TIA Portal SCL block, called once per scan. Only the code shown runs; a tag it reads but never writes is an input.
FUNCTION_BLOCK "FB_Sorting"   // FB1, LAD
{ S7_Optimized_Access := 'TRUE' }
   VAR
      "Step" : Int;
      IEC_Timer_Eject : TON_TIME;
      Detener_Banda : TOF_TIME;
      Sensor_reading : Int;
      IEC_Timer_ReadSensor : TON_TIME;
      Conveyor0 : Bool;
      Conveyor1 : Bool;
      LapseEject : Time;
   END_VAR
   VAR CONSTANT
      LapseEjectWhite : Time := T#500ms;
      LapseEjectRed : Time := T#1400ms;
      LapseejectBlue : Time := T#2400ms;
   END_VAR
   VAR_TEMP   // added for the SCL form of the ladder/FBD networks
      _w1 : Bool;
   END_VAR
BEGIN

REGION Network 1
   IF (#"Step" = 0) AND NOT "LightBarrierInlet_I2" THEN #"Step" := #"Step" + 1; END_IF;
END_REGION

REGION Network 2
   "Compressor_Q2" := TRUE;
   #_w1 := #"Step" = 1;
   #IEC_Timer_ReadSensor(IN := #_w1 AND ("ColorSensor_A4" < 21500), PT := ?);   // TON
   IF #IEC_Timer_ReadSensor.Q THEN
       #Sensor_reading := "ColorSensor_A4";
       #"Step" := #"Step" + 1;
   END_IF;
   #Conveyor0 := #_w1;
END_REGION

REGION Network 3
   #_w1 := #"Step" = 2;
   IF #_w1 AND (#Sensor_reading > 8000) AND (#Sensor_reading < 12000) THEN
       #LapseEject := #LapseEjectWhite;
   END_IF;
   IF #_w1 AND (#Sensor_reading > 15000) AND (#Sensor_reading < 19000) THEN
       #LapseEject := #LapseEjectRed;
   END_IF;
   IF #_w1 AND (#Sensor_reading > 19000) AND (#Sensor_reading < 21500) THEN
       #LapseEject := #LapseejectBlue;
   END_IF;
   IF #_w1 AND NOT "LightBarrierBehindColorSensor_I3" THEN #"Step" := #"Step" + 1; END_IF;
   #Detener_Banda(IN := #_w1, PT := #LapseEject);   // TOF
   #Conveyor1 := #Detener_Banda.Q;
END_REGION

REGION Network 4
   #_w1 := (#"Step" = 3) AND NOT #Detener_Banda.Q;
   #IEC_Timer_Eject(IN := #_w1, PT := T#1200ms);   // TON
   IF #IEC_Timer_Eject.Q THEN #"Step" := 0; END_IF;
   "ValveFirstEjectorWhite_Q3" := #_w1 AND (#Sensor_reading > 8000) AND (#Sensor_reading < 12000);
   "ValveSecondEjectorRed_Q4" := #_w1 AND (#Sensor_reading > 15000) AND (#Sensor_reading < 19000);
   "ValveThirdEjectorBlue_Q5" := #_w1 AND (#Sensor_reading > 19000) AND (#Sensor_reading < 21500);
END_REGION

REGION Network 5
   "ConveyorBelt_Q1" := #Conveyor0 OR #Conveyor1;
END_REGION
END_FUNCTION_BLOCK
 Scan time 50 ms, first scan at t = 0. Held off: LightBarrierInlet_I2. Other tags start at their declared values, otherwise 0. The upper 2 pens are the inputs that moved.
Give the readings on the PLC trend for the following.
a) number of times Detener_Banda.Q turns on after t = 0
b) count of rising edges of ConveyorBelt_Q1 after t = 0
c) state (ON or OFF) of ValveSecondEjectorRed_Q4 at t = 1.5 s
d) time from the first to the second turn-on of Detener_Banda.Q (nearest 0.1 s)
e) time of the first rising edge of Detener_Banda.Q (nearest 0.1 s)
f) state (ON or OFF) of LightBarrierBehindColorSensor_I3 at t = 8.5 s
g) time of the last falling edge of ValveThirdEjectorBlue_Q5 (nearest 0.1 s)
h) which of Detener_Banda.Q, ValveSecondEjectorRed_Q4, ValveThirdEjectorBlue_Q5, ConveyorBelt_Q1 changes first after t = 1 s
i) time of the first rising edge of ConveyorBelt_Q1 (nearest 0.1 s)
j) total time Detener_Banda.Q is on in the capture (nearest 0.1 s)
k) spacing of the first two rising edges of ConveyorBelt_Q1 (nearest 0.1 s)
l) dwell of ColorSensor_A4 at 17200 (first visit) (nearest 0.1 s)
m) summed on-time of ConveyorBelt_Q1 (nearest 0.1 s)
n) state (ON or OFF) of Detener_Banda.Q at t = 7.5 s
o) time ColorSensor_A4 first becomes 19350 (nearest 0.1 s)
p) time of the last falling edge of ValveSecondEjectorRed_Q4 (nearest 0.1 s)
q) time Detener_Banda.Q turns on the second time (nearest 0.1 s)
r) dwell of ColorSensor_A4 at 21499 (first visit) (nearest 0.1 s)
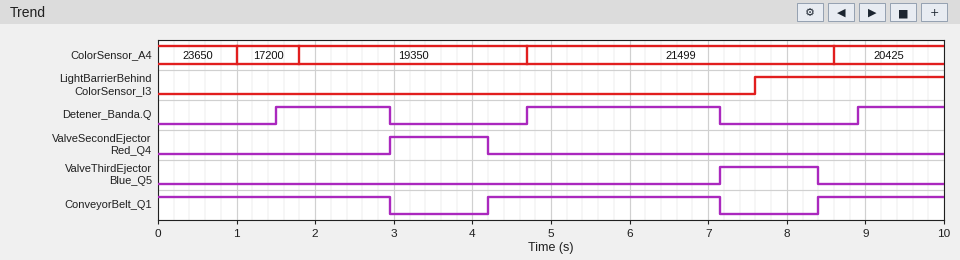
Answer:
3
2
OFF
3.2 s
1.5 s
ON
8.4 s
Detener_Banda.Q
4.2 s
5.0 s
4.2 s
0.8 s
7.5 s
OFF
1.8 s
4.2 s
4.7 s
3.9 s
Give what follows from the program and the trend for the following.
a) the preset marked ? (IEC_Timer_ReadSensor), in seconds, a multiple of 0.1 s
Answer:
0.5 s
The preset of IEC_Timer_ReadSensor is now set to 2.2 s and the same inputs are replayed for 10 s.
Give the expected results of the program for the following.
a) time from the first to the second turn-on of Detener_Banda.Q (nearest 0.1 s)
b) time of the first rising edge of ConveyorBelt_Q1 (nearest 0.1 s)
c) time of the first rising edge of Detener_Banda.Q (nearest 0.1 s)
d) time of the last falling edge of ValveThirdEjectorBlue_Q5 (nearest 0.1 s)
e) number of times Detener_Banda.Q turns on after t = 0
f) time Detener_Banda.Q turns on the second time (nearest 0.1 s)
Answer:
5.9 s
6.9 s
3.2 s
6.9 s
2
9.1 s
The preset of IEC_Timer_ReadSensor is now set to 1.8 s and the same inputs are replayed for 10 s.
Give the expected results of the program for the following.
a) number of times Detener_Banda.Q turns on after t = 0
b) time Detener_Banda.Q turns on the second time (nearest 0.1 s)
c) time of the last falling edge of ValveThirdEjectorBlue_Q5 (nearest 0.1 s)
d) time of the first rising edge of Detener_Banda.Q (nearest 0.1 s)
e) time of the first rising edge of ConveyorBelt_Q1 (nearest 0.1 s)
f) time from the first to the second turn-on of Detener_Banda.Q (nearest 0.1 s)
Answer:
2
8.3 s
6.5 s
2.8 s
6.5 s
5.5 s
